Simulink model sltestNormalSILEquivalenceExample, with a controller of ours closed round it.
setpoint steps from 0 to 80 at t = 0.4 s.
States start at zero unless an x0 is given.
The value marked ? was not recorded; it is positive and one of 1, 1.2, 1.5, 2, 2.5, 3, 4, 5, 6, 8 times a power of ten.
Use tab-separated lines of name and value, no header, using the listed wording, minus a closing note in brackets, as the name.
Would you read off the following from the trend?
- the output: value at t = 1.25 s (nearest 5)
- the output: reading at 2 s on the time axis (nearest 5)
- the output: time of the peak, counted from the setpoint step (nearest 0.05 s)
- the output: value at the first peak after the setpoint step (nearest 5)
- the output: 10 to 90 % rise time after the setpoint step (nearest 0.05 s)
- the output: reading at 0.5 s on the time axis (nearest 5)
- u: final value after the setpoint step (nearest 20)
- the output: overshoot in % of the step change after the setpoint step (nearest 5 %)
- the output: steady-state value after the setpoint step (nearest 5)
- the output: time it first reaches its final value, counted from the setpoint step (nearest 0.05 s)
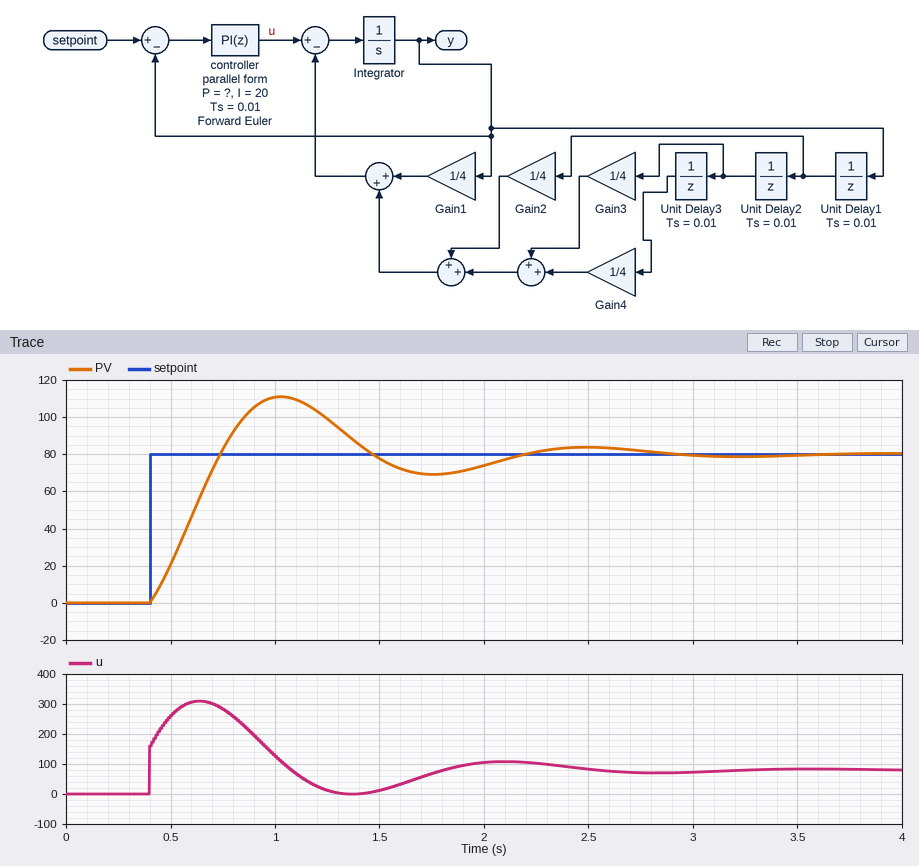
the output: value at t = 1.25 s	100
the output: reading at 2 s on the time axis	75
the output: time of the peak, counted from the setpoint step	0.65 s
the output: value at the first peak after the setpoint step	110
the output: 10 to 90 % rise time after the setpoint step	0.25 s
the output: reading at 0.5 s on the time axis	20
u: final value after the setpoint step	80
the output: overshoot in % of the step change after the setpoint step	40 %
the output: steady-state value after the setpoint step	80
the output: time it first reaches its final value, counted from the setpoint step	0.35 s
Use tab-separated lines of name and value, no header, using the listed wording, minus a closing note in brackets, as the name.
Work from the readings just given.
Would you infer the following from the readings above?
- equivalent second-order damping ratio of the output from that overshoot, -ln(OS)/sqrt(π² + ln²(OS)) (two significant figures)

equivalent second-order damping ratio of the output from that overshoot, -ln(OS)/sqrt(π² + ln²(OS))	0.28
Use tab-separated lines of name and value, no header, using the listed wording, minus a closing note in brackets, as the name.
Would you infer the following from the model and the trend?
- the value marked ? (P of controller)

the value marked ?	2
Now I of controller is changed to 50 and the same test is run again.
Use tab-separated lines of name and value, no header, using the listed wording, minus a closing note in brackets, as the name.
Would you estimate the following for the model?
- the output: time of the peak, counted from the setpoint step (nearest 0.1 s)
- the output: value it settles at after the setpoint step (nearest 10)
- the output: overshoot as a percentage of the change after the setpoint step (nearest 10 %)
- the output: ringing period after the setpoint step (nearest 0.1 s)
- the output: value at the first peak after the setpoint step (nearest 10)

the output: time of the peak, counted from the setpoint step	0.4 s
the output: value it settles at after the setpoint step	80
the output: overshoot as a percentage of the change after the setpoint step	60 %
the output: ringing period after the setpoint step	0.9 s
the output: value at the first peak after the setpoint step	130
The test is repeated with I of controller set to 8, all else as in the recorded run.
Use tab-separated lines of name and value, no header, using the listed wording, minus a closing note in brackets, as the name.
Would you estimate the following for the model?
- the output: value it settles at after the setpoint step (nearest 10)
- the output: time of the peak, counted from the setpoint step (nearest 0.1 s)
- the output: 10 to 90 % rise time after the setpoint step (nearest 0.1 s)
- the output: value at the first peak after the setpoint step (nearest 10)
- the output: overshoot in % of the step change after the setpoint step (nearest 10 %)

the output: value it settles at after the setpoint step	80
the output: time of the peak, counted from the setpoint step	1.0 s
the output: 10 to 90 % rise time after the setpoint step	0.4 s
the output: value at the first peak after the setpoint step	100
the output: overshoot in % of the step change after the setpoint step	20 %
